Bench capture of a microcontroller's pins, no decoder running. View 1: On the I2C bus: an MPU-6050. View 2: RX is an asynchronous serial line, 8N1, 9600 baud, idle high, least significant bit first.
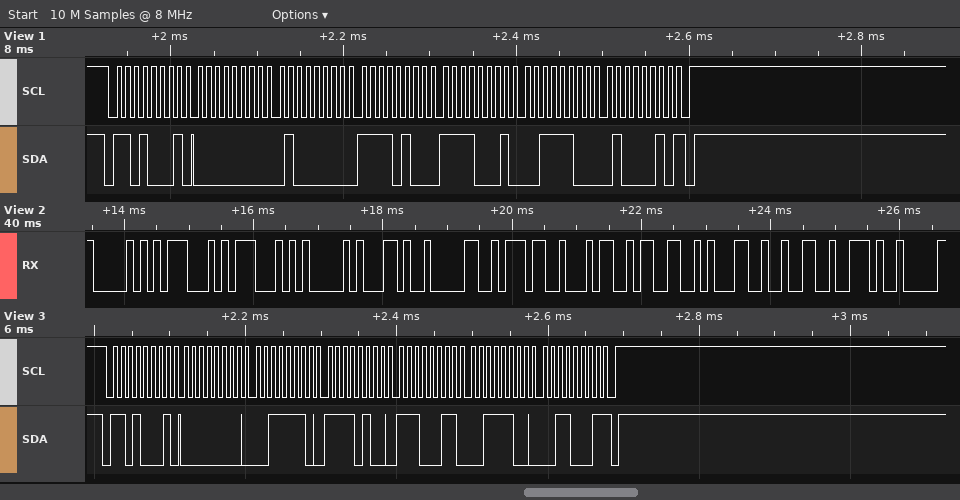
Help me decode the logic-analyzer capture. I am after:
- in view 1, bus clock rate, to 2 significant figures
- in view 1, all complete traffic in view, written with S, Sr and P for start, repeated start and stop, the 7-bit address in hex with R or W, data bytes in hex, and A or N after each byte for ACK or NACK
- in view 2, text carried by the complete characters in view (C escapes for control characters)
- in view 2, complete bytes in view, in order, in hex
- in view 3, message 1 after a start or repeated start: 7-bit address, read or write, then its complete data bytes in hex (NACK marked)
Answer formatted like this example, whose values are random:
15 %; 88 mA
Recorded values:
100 kHz; S 68R A 00 A 40 A F4 A F1 A 3C A 42 N P; "PGGA,074312."; 50 47 47 41 2C 30 37 34 33 31 32 2E; 0x68 read: 00 3E F4 E3 3C 31 NACK
